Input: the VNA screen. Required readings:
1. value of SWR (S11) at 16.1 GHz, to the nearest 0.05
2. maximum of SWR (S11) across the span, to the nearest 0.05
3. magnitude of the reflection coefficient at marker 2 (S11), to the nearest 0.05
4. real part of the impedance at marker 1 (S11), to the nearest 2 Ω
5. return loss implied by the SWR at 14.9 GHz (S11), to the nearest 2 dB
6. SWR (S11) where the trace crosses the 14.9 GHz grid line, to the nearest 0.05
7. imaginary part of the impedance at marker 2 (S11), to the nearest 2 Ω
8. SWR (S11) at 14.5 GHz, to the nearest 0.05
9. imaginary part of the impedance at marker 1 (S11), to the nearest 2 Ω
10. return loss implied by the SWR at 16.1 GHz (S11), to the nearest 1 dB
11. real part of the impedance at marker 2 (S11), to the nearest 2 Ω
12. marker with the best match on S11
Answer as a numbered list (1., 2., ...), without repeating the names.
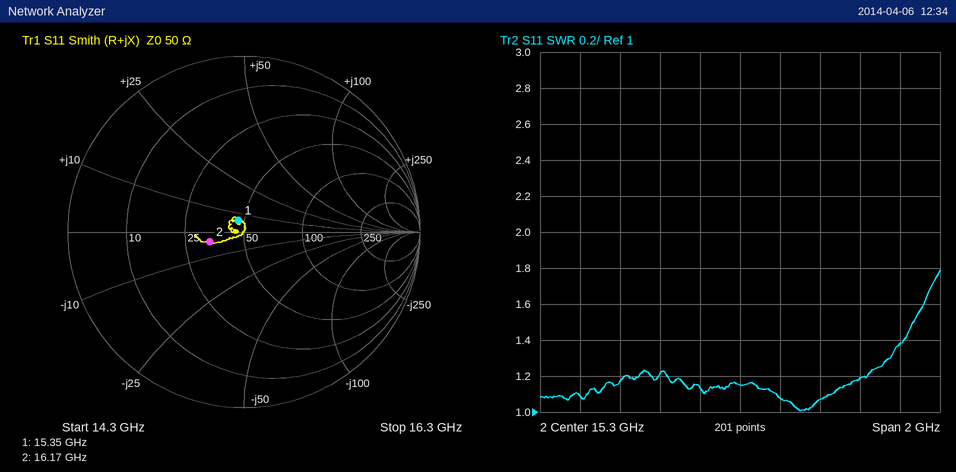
1. 1.40
2. 1.80
3. 0.20
4. 46 Ω
5. 20 dB
6. 1.20
7. -4 Ω
8. 1.10
9. +6 Ω
10. 16 dB
11. 34 Ω
12. marker 1
